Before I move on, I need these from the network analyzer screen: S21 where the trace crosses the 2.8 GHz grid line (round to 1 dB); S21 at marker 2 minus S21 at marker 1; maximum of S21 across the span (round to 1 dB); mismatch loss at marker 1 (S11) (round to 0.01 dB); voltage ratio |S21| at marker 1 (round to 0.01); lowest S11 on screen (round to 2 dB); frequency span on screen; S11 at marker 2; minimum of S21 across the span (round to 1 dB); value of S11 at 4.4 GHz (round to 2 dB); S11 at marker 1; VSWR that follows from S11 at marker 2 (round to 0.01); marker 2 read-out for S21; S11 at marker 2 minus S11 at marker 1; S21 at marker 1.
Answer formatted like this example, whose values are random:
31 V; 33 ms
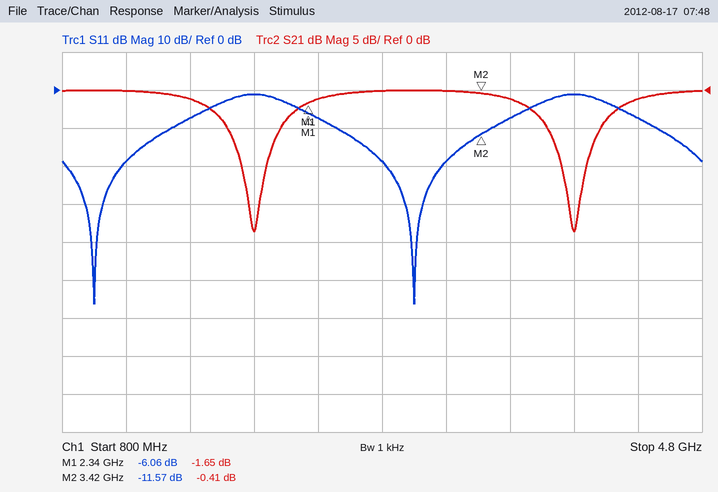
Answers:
0 dB; 1.24 dB; 0 dB; 1.24 dB; 0.83; -56 dB; 4 GHz; -11.57 dB; -19 dB; -8 dB; -6.06 dB; 1.72; -0.41 dB; -5.51 dB; -1.65 dB
